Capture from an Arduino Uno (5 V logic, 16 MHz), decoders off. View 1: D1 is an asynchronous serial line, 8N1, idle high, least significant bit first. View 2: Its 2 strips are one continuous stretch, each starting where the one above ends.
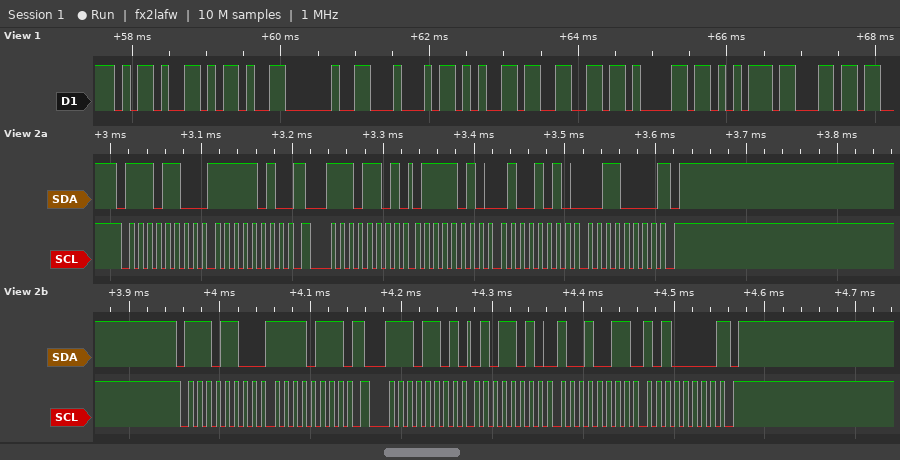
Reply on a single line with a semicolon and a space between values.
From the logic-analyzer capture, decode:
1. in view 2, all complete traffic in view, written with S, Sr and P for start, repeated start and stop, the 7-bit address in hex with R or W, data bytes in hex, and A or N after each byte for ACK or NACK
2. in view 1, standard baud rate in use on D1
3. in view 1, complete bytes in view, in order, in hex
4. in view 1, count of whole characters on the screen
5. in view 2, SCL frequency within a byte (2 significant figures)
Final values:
S 76W A FA A Sr 76R A 7A A 4A A 30 N P S 76W A F7 A Sr 76R A 5A A 93 A A0 N P; 9600 baud; 2D 2D 20 44 65 66 61 75 6C; 9; 100 kHz
